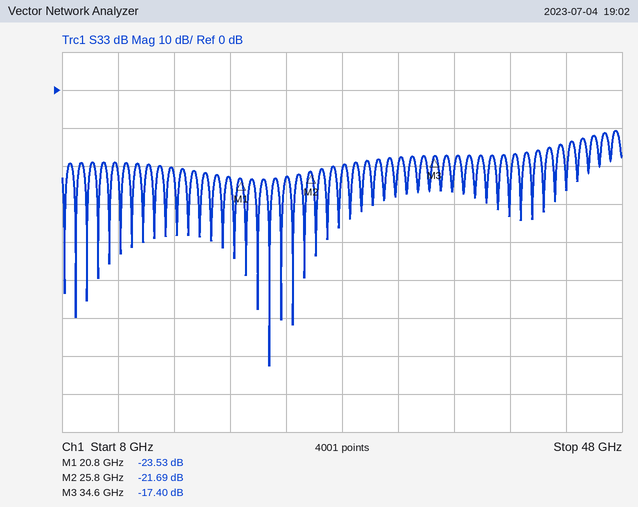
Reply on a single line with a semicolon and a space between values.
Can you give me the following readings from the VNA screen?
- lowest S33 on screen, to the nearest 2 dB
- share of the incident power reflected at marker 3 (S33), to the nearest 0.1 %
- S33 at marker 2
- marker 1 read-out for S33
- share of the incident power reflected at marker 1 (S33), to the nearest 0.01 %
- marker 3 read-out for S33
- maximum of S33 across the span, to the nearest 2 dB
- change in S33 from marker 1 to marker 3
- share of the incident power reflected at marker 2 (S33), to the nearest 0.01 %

-72 dB; 1.8 %; -21.69 dB; -23.53 dB; 0.44 %; -17.40 dB; -10 dB; 6.13 dB; 0.68 %
